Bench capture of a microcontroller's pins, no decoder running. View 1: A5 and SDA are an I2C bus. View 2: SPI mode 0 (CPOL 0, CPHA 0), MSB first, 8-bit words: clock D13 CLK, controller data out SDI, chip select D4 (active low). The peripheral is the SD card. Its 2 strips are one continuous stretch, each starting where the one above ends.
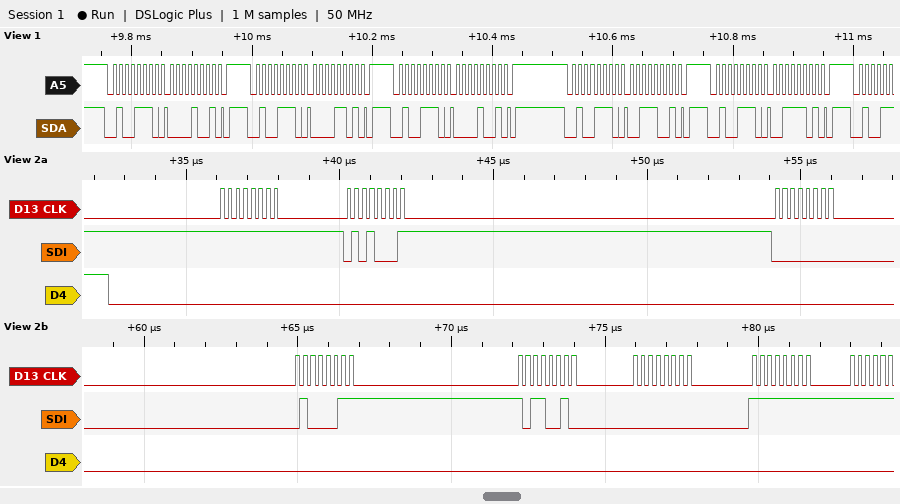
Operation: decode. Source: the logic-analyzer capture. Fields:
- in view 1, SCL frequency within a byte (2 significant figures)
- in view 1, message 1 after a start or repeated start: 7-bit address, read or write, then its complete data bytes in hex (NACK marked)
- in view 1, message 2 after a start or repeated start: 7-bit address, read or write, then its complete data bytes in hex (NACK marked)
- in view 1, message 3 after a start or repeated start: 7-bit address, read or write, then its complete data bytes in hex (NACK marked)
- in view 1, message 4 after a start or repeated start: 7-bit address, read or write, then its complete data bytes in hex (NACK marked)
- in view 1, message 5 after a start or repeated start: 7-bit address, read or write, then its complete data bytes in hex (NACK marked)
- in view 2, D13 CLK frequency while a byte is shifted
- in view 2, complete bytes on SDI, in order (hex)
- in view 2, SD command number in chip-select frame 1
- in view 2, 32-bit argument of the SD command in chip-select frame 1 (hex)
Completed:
100 kHz
0x27 write: 09
0x27 write: 0D
0x27 write: 09
0x27 write: 39
0x27 write: 3D
4 MHz
FF 51 00 43 B2 00 FF
CMD17
0x0043B200
